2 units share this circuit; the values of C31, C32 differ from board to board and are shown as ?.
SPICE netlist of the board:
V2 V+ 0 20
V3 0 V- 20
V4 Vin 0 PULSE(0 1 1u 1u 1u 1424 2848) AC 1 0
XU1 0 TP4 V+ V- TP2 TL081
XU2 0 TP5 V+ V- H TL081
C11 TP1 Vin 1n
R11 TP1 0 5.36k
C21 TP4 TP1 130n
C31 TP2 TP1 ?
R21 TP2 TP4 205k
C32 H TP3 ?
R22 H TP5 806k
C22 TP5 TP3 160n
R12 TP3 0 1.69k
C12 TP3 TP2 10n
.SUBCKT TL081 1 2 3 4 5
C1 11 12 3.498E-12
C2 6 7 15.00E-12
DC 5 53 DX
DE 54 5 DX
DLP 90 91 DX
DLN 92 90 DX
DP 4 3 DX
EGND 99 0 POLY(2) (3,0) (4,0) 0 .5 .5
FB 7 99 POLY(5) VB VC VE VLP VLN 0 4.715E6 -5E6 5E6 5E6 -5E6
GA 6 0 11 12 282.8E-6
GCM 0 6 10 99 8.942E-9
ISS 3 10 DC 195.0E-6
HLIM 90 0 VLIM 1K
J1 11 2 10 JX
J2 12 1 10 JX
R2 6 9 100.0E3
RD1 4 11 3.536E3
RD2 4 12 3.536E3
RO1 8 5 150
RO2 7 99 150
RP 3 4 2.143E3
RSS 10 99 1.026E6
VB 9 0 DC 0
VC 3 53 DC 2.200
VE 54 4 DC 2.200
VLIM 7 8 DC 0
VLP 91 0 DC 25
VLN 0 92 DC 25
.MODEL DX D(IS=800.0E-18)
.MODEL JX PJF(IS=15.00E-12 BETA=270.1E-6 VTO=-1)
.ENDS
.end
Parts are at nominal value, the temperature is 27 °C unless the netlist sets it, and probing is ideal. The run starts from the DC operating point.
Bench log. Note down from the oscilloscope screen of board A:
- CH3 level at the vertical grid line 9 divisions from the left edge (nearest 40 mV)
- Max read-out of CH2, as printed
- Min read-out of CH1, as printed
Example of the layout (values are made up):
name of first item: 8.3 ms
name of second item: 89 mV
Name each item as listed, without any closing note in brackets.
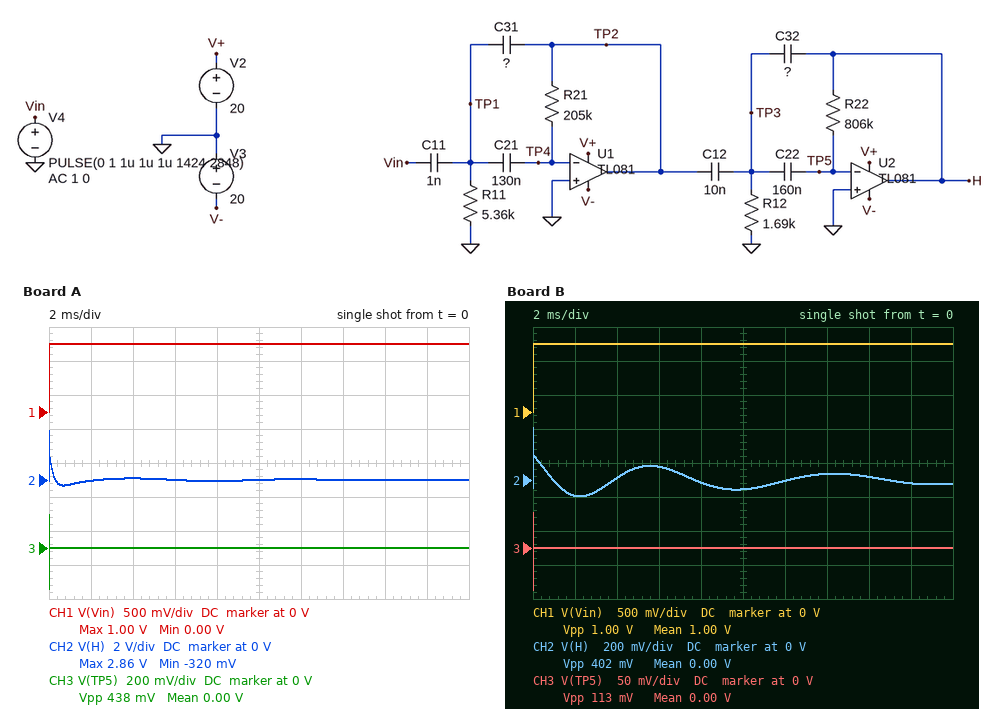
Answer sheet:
CH3 level at the vertical grid line 9 divisions from the left edge: 0 V
Max read-out of CH2, as printed: 2.86 V
Min read-out of CH1, as printed: 0.00 V
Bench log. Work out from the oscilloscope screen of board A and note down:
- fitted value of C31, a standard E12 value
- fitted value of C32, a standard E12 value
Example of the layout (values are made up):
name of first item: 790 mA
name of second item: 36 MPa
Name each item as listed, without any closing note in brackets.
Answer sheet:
fitted value of C31, a standard E12 value: 820 pF
fitted value of C32, a standard E12 value: 6.8 nF
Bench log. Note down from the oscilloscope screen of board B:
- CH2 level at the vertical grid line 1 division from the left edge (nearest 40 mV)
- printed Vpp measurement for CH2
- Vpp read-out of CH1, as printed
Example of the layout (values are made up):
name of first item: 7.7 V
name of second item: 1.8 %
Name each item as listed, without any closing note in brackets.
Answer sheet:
CH2 level at the vertical grid line 1 division from the left edge: -80 mV
printed Vpp measurement for CH2: 402 mV
Vpp read-out of CH1, as printed: 1.00 V
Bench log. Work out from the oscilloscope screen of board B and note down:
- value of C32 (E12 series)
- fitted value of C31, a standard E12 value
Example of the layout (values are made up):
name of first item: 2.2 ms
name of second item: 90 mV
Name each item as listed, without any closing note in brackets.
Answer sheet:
value of C32: 10 nF
fitted value of C31, a standard E12 value: 6.8 nF
